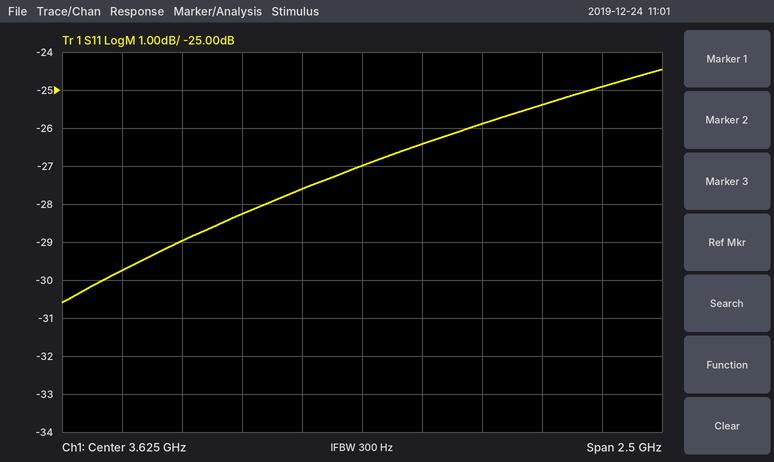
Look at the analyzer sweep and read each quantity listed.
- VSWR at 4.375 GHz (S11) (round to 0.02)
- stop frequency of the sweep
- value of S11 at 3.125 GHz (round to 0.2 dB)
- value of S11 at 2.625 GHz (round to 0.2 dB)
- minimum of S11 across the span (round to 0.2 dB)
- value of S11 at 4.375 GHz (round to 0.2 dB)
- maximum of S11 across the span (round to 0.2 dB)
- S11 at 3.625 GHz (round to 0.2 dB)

1.12
4.875 GHz
-28.2 dB
-29.8 dB
-30.6 dB
-25.4 dB
-24.4 dB
-27.0 dB
